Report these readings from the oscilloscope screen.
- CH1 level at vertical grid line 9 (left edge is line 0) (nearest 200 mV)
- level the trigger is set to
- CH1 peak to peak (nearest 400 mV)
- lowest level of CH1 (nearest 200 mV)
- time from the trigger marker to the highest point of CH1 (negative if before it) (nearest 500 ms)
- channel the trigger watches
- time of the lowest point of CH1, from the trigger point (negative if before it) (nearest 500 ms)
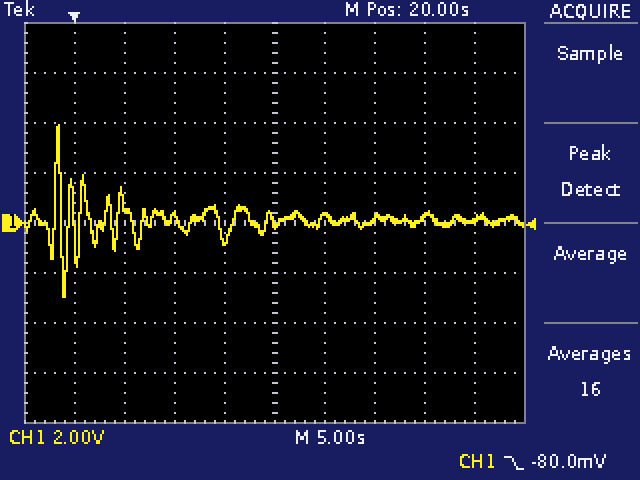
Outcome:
200 mV
-80.0 mV
6.8 V
-3.0 V
-1.5 s
CH1
-1.0 s
